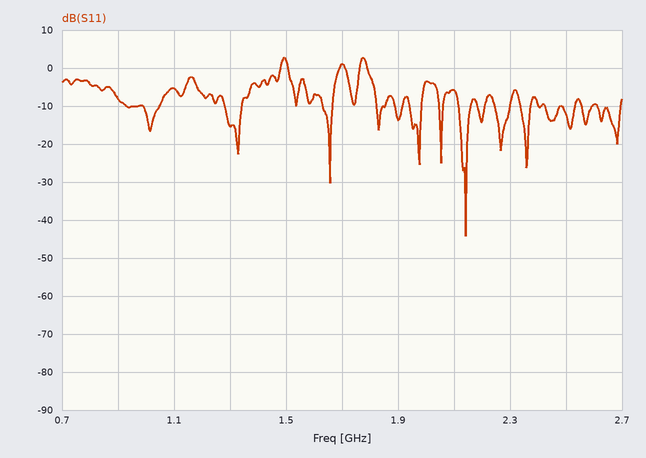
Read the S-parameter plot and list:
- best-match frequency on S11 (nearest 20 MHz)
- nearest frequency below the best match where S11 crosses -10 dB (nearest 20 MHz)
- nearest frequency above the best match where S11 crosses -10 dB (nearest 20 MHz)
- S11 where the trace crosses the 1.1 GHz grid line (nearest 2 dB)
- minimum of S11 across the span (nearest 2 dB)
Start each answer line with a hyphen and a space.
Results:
- 2.14 GHz
- 2.12 GHz
- 2.16 GHz
- -6 dB
- -44 dB
